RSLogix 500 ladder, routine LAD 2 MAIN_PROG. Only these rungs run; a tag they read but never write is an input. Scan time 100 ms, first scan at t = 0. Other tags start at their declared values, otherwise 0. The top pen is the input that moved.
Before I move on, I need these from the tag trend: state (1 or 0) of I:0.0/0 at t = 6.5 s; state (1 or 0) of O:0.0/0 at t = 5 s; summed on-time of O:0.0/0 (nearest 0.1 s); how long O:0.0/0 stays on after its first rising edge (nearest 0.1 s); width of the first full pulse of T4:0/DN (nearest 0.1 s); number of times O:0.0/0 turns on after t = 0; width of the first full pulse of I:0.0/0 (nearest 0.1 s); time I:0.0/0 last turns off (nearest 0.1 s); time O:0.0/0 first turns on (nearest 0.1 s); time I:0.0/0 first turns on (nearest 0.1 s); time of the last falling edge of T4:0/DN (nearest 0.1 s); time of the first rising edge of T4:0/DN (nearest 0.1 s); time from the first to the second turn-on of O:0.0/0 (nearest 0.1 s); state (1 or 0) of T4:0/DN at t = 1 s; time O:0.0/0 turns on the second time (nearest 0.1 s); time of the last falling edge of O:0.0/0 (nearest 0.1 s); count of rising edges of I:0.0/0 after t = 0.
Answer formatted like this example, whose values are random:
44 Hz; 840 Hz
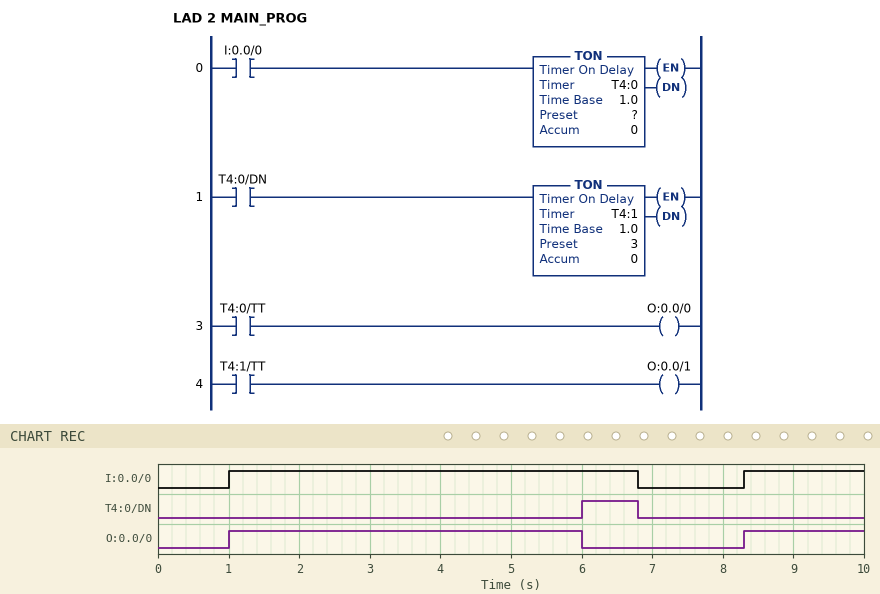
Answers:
1; 1; 6.7 s; 5.0 s; 0.8 s; 2; 5.8 s; 6.8 s; 1.0 s; 1.0 s; 6.8 s; 6.0 s; 7.3 s; 0; 8.3 s; 6.0 s; 2
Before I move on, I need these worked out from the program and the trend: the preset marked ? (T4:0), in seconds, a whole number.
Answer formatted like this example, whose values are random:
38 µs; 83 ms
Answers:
5 s
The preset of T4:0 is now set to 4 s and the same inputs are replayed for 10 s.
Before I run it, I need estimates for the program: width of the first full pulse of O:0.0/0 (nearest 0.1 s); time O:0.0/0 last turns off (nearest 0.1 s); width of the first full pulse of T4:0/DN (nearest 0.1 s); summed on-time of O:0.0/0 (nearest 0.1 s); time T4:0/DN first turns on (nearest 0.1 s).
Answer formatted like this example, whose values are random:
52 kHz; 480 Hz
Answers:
4.0 s; 5.0 s; 1.8 s; 5.7 s; 5.0 s
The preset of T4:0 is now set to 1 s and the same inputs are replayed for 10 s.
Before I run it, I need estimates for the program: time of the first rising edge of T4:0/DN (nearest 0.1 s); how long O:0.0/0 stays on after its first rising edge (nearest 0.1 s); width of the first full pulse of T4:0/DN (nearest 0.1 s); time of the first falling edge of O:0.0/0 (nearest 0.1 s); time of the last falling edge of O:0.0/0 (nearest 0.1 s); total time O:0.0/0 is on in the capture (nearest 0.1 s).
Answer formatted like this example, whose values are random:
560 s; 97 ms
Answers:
2.0 s; 1.0 s; 4.8 s; 2.0 s; 9.3 s; 2.0 s
